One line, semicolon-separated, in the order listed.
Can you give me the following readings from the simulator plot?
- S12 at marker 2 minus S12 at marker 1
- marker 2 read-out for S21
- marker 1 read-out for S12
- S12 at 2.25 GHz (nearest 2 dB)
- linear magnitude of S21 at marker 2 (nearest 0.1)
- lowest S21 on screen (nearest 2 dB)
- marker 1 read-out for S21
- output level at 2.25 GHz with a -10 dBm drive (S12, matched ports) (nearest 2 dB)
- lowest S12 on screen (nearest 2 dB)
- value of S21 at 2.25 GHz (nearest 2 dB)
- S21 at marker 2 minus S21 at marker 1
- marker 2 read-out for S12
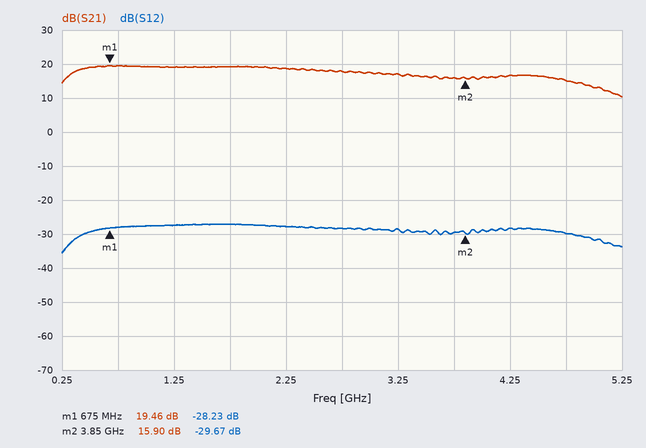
-1.44 dB; 15.90 dB; -28.23 dB; -28 dB; 6.2; 10 dB; 19.46 dB; -38 dBm; -36 dB; 18 dB; -3.56 dB; -29.67 dB
